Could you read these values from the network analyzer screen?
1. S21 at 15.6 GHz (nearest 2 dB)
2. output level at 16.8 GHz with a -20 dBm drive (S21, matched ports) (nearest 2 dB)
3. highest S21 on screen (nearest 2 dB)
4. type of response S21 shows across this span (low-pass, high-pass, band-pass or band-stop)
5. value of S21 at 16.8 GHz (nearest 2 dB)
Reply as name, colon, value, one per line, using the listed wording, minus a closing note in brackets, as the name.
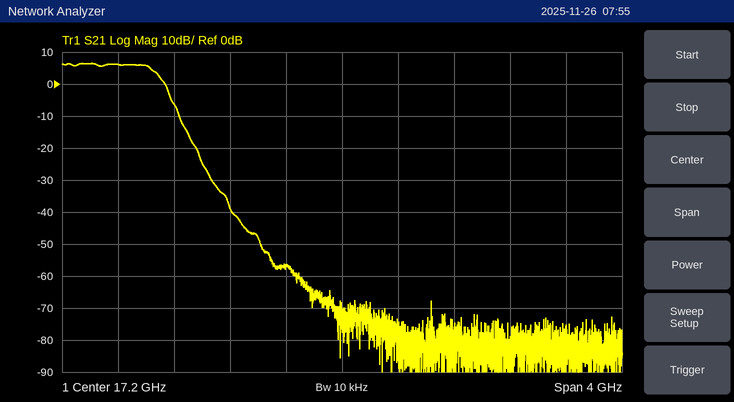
S21 at 15.6 GHz: 6 dB
output level at 16.8 GHz with a -20 dBm drive (S21, matched ports): -76 dBm
highest S21 on screen: 6 dB
type of response S21 shows across this span: low-pass
value of S21 at 16.8 GHz: -56 dB
